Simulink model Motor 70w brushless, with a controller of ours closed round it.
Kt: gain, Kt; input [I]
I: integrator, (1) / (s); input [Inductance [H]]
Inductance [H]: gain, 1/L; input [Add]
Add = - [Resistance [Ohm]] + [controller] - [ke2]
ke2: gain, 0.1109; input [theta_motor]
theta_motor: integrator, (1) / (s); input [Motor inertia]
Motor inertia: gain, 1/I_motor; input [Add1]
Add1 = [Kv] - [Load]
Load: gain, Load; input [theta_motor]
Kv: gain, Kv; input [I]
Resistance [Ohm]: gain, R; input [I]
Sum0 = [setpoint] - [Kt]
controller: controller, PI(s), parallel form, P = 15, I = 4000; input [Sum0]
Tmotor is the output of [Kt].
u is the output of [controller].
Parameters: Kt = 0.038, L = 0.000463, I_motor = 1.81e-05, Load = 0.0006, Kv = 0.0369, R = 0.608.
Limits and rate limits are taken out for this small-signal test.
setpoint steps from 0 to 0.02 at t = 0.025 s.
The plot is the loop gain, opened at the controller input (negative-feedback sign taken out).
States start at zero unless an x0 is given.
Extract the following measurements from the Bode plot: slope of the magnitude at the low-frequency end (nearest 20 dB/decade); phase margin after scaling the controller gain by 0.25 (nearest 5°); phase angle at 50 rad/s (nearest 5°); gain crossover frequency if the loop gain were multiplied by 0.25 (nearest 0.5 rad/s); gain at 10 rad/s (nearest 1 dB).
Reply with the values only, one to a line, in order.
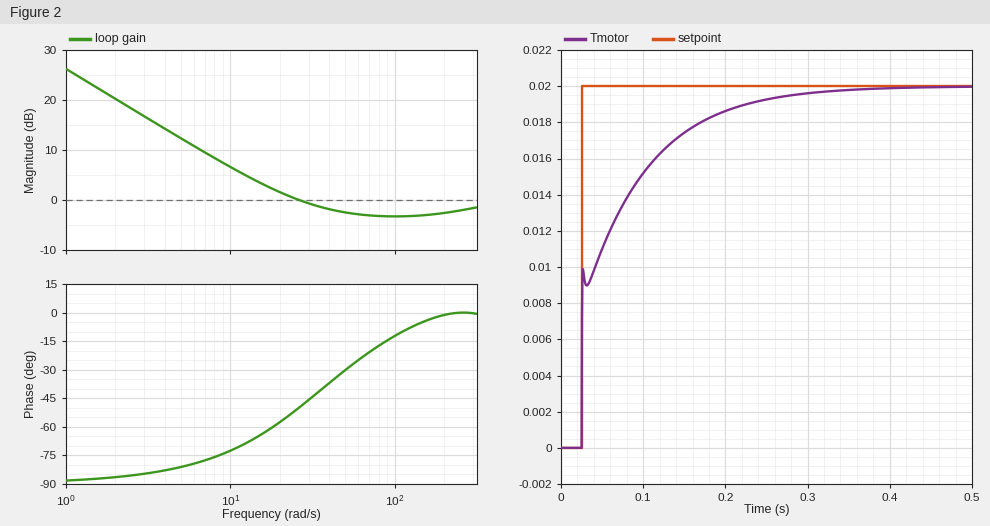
-20 dB/decade
100°
-30°
5.0 rad/s
7 dB
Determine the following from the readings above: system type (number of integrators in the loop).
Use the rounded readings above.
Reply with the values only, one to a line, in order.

1
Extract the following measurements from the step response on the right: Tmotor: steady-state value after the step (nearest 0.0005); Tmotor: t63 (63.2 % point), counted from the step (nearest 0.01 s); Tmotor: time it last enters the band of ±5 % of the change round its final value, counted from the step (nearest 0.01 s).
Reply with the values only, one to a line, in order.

0.0200
0.04 s
0.20 s
